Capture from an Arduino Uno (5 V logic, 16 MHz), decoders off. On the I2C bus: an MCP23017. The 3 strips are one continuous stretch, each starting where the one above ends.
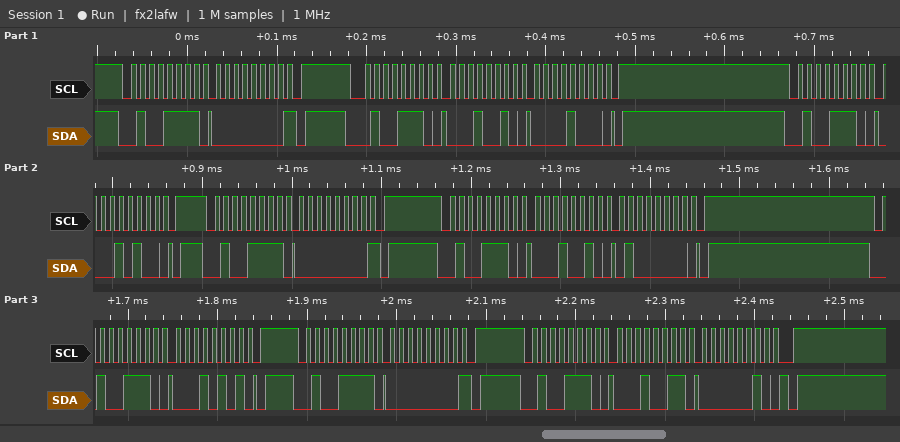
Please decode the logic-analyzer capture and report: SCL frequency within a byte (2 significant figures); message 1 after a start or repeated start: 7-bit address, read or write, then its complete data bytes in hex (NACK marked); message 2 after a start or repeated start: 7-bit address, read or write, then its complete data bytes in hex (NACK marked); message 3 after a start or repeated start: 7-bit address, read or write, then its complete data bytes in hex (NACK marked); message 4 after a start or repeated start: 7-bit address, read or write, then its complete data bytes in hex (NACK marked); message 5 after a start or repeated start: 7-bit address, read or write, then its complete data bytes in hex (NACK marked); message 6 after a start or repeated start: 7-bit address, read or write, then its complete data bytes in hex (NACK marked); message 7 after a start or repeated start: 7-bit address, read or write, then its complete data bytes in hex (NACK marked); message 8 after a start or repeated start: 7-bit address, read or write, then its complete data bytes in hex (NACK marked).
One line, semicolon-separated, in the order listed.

100 kHz; 0x27 read: 00 NACK; 0x27 write: 12 08; 0x27 write: 14; 0x27 read: 00 NACK; 0x27 write: 12 40; 0x27 write: 15; 0x27 read: 00 NACK; 0x27 write: 13 02
